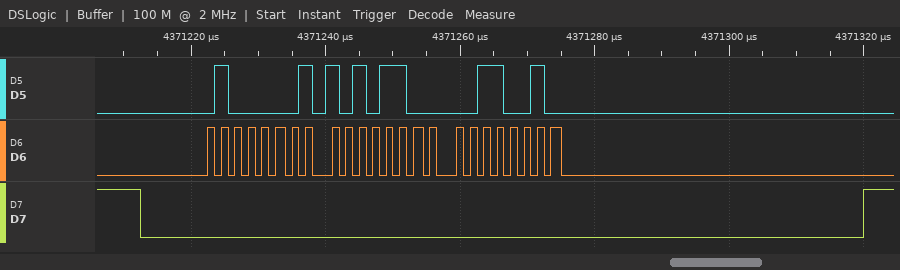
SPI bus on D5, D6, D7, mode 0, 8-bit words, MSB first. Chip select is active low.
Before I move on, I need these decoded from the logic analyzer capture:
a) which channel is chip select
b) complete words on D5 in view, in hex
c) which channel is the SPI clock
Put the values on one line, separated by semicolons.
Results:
D7; 41, AC, 32; D6
